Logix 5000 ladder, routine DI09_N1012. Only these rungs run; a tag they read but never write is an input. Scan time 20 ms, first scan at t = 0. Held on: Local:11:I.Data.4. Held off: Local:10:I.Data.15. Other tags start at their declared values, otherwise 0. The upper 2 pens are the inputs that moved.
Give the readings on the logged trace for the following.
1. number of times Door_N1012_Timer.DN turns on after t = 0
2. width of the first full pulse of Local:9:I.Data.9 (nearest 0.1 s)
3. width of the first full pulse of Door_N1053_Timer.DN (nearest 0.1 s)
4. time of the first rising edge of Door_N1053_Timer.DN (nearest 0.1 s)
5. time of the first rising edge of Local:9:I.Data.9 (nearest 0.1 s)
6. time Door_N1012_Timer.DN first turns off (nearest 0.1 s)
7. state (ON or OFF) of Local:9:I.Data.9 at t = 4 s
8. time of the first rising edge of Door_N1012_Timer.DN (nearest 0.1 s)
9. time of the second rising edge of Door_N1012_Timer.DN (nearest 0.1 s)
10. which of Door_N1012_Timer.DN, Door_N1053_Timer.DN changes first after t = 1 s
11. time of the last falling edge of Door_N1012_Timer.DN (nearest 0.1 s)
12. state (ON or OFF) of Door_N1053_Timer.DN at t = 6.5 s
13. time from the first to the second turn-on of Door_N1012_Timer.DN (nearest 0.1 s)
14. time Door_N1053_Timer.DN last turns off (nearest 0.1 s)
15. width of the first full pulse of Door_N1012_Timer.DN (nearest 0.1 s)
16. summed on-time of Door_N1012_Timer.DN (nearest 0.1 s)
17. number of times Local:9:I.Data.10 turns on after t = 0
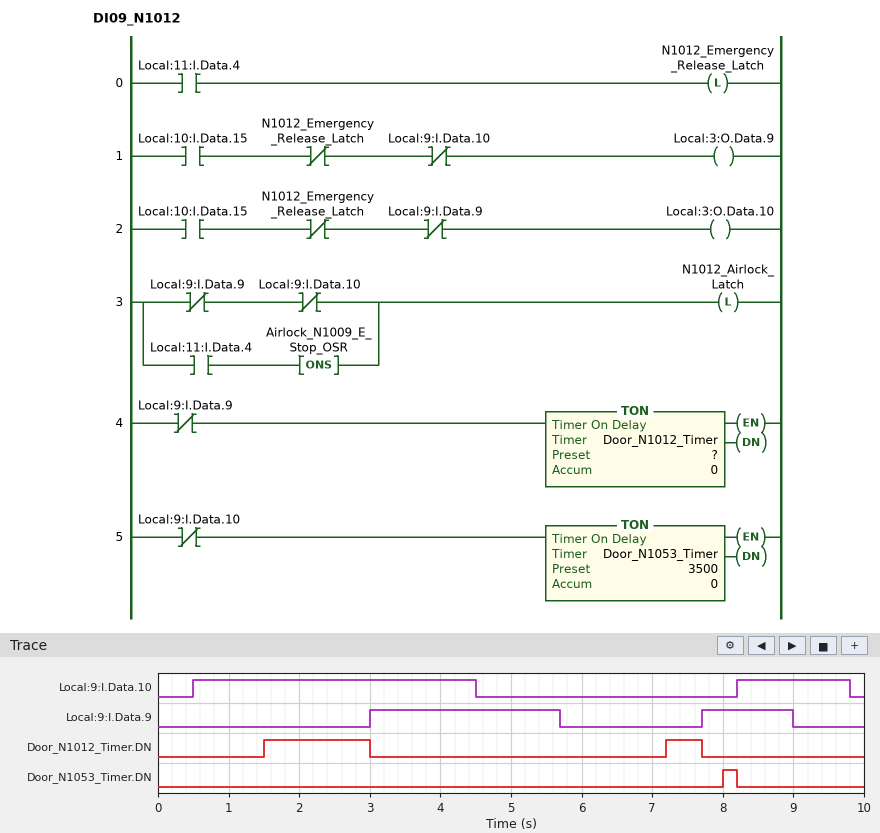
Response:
2
2.7 s
0.2 s
8.0 s
3.0 s
3.0 s
ON
1.5 s
7.2 s
Door_N1012_Timer.DN
7.7 s
OFF
5.7 s
8.2 s
1.5 s
2.0 s
2
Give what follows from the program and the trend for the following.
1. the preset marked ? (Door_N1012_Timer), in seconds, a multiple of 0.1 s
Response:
1.5 s
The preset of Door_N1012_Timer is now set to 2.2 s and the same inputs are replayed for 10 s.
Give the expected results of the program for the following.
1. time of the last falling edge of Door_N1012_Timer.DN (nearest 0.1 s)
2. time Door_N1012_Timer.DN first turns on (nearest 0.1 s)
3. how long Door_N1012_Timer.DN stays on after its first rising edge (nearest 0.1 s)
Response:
3.0 s
2.2 s
0.8 s
